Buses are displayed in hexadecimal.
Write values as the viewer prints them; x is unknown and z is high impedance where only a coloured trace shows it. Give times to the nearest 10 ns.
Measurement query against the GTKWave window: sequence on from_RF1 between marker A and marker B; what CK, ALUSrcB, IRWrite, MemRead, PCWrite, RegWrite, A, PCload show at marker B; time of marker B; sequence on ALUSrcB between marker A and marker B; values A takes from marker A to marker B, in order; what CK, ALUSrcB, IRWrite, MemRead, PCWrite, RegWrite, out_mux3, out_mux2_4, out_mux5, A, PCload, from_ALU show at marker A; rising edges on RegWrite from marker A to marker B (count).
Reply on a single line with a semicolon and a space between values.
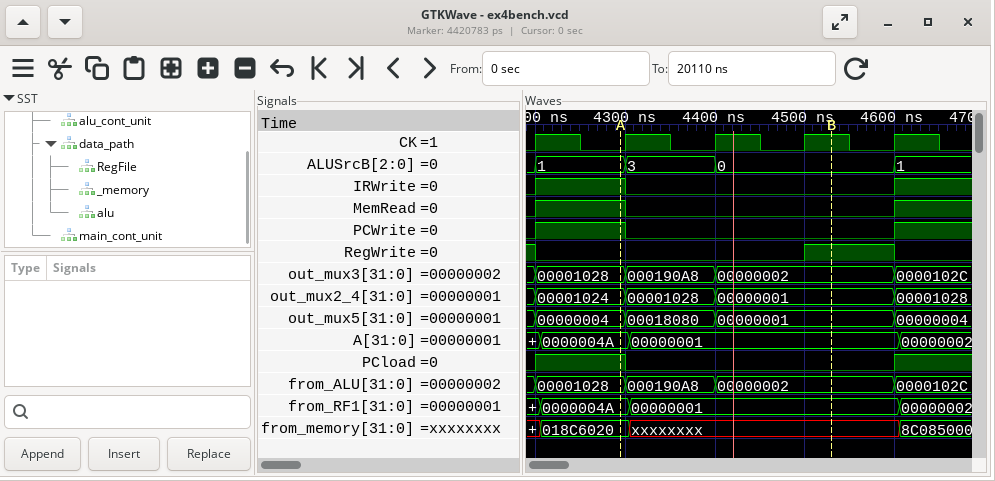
0000004A, 00000001; CK=1, ALUSrcB=0, IRWrite=0, MemRead=0, PCWrite=0, RegWrite=1, A=00000001, PCload=0; 4530 ns; 1, 3, 0; 0000004A, 00000001; CK=0, ALUSrcB=1, IRWrite=1, MemRead=1, PCWrite=1, RegWrite=0, out_mux3=00001028, out_mux2_4=00001024, out_mux5=00000004, A=0000004A, PCload=1, from_ALU=00001028; 1
